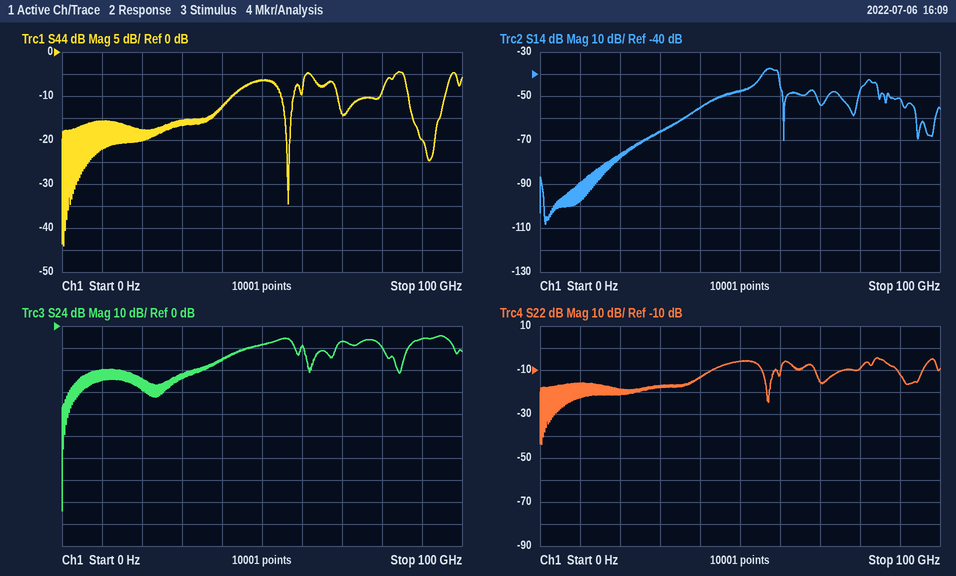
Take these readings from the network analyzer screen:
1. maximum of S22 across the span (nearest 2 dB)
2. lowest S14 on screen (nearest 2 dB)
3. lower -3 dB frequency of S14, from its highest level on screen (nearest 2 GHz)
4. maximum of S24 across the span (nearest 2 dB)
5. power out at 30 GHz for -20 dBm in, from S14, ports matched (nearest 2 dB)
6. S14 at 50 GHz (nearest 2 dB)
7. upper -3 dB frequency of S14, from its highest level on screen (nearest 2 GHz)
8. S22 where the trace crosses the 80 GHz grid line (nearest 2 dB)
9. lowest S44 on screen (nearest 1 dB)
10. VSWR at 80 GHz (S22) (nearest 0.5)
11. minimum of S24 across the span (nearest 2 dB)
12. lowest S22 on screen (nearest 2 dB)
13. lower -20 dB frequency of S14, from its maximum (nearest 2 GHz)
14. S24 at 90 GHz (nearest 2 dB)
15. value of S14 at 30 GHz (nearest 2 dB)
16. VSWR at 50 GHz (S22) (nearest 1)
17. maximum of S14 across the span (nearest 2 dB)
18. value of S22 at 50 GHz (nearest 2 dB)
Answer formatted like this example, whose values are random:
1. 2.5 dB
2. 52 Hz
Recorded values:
1. -4 dB
2. -108 dB
3. 56 GHz
4. -4 dB
5. -86 dBm
6. -48 dB
7. 60 GHz
8. -10 dB
9. -44 dB
10. 2.0
11. -84 dB
12. -44 dB
13. 38 GHz
14. -6 dB
15. -66 dB
16. 3
17. -38 dB
18. -6 dB
